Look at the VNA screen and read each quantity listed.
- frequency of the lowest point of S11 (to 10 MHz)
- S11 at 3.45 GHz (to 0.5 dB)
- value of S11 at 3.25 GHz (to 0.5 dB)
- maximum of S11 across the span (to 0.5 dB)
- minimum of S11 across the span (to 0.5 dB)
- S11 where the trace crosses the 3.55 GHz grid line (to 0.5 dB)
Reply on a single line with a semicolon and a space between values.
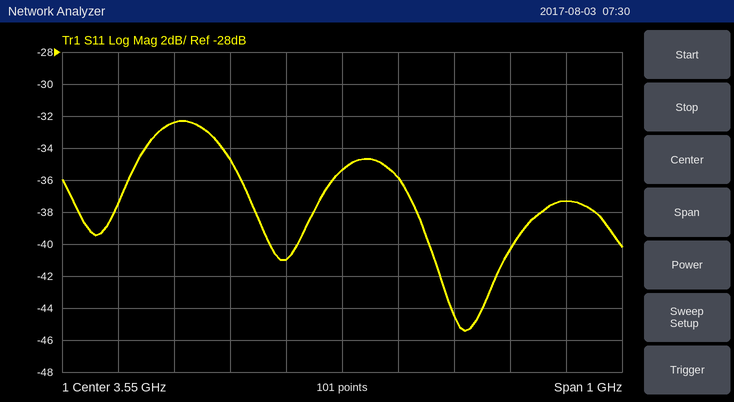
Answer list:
3.77 GHz; -41.0 dB; -32.5 dB; -32.5 dB; -45.5 dB; -35.5 dB
